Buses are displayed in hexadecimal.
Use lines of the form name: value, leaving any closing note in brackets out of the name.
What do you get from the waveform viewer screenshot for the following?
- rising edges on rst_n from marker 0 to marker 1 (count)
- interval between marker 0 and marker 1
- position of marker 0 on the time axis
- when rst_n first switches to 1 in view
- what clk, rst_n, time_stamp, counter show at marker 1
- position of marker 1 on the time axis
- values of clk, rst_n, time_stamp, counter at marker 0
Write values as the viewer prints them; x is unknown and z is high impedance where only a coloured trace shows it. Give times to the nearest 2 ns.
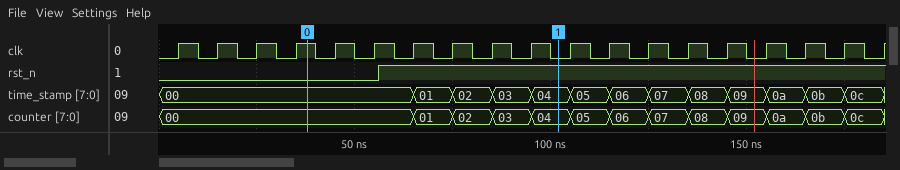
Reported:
rising edges on rst_n from marker 0 to marker 1: 1
interval between marker 0 and marker 1: 64 ns
position of marker 0 on the time axis: 38 ns
when rst_n first switches to 1 in view: 56 ns
what clk, rst_n, time_stamp, counter show at marker 1: clk=0, rst_n=1, time_stamp=04, counter=04
position of marker 1 on the time axis: 102 ns
values of clk, rst_n, time_stamp, counter at marker 0: clk=1, rst_n=0, time_stamp=00, counter=00
